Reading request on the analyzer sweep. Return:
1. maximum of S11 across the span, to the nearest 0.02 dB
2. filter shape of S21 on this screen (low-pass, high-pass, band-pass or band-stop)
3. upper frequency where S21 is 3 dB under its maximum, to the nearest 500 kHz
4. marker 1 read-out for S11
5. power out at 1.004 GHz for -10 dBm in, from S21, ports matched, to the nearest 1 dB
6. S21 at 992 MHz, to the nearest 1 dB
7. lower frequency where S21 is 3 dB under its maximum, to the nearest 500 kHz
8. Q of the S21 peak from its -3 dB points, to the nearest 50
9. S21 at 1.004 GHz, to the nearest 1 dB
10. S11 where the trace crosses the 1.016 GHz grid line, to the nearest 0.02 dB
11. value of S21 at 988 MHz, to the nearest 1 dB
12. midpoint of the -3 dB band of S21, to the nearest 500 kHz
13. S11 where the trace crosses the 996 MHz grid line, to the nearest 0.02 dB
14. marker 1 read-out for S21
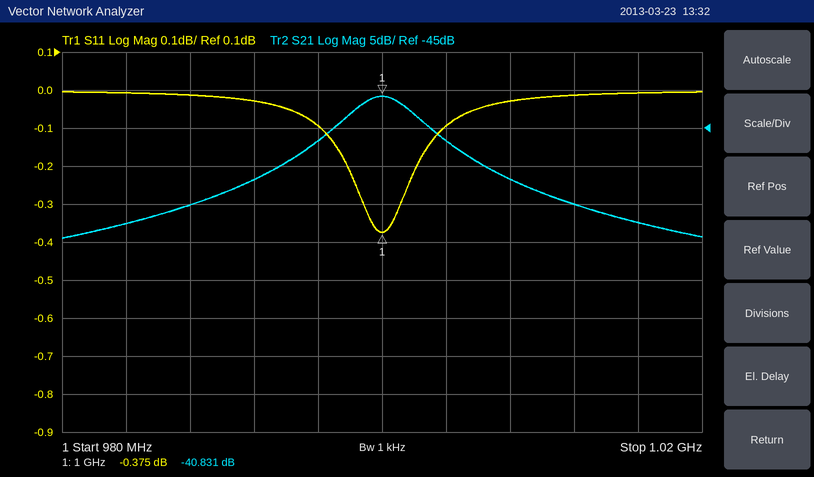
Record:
0.00 dB
band-pass
1.0025 GHz
-0.375 dB
-57 dBm
-52 dB
997.5 MHz
200
-47 dB
0.00 dB
-55 dB
1.0000 GHz
-0.10 dB
-40.831 dB
